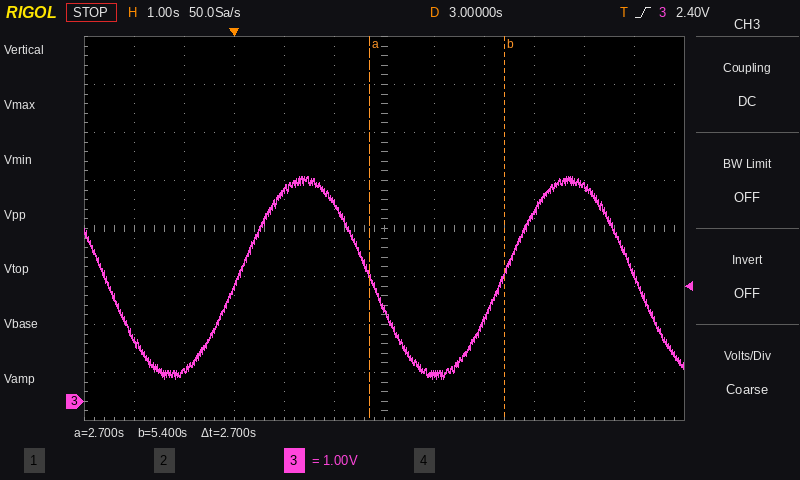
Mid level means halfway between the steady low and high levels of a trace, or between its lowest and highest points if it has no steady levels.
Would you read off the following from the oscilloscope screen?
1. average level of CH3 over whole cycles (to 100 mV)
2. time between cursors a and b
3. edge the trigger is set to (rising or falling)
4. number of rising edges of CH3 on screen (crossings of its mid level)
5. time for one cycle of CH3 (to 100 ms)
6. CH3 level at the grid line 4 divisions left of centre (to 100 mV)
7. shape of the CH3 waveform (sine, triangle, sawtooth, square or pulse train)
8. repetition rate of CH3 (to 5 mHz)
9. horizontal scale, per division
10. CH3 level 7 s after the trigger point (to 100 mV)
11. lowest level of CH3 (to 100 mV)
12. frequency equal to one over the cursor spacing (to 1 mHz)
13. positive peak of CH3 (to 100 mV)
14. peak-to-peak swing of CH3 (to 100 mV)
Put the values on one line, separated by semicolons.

2.6 V; 2.7 s; rising; 2; 5.3 s; 700 mV; sine; 190 mHz; 1 s; 4.5 V; 500 mV; 370 mHz; 4.7 V; 4.2 V
